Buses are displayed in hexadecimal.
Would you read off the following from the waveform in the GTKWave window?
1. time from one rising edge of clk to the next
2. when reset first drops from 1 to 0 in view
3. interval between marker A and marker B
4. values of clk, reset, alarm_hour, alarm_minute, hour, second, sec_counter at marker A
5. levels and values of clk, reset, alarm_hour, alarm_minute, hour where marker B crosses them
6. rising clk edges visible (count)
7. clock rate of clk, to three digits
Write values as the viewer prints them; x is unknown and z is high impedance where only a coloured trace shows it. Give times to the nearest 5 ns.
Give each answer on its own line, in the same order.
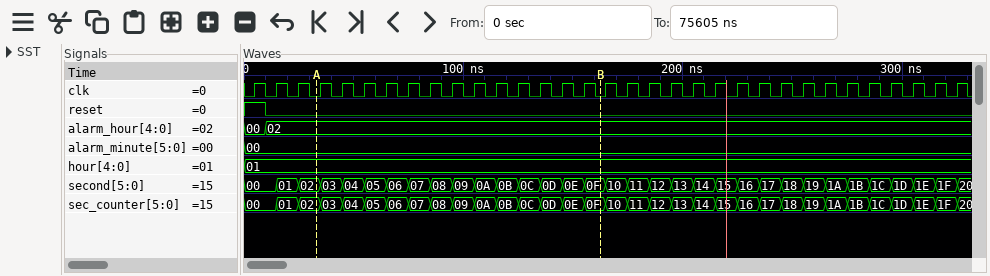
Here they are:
10 ns
10 ns
130 ns
clk=0, reset=0, alarm_hour=02, alarm_minute=00, hour=01, second=02, sec_counter=02
clk=0, reset=0, alarm_hour=02, alarm_minute=00, hour=01
33
100 MHz
